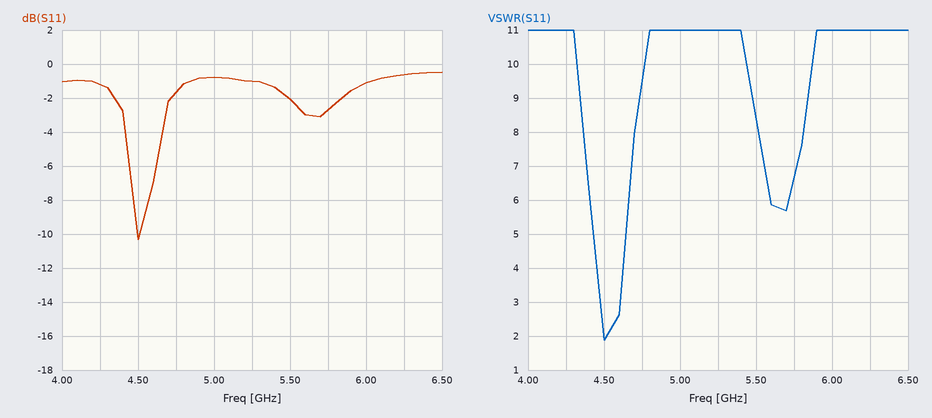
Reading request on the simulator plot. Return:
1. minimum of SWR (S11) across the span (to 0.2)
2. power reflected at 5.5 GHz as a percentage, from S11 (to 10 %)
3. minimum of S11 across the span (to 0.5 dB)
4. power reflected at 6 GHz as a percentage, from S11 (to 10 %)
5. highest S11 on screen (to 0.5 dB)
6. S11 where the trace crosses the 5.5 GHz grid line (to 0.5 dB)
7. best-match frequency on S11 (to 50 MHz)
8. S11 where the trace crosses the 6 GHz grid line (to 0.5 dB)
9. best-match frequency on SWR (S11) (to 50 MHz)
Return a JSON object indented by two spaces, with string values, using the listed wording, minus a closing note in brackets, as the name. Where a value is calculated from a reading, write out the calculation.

{
  "minimum of SWR (S11) across the span": "1.8",
  "power reflected at 5.5 GHz as a percentage, from S11": "10^(-2/10) ≈ 63.1 %, so 60 % to the nearest 10 %",
  "minimum of S11 across the span": "-10.5 dB",
  "power reflected at 6 GHz as a percentage, from S11": "10^(-1/10) ≈ 79.4 %, so 80 % to the nearest 10 %",
  "highest S11 on screen": "-0.5 dB",
  "S11 where the trace crosses the 5.5 GHz grid line": "-2.0 dB",
  "best-match frequency on S11": "4.50 GHz",
  "S11 where the trace crosses the 6 GHz grid line": "-1.0 dB",
  "best-match frequency on SWR (S11)": "4.50 GHz"
}
